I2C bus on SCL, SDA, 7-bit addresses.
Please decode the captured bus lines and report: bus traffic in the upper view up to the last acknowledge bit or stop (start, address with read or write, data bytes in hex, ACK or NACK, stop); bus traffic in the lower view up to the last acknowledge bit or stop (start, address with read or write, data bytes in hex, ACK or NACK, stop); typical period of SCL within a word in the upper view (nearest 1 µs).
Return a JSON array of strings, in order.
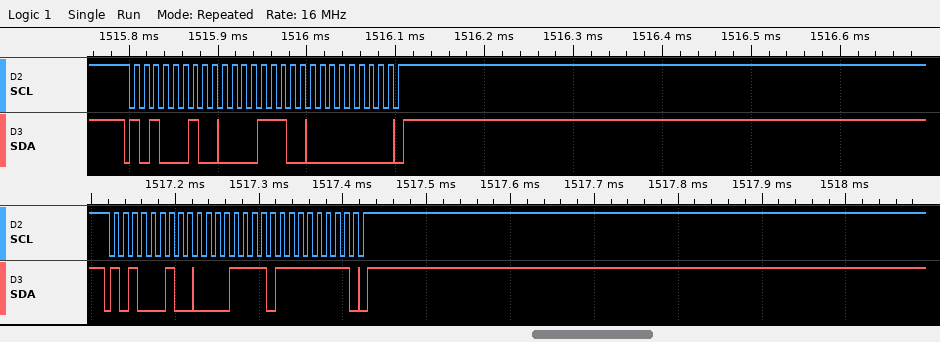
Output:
["start, address 51 write ACK, 0E ACK, 00 ACK, stop", "start, address 51 write ACK, 0F ACK, FF ACK, stop", "11 µs"]
